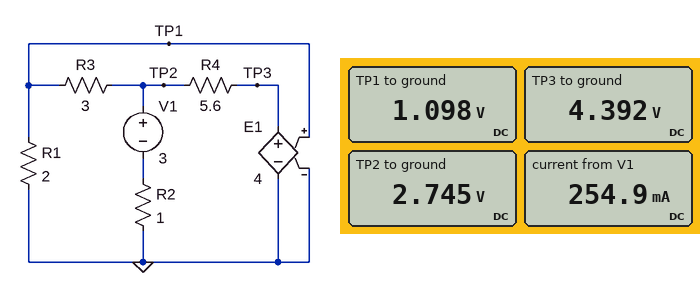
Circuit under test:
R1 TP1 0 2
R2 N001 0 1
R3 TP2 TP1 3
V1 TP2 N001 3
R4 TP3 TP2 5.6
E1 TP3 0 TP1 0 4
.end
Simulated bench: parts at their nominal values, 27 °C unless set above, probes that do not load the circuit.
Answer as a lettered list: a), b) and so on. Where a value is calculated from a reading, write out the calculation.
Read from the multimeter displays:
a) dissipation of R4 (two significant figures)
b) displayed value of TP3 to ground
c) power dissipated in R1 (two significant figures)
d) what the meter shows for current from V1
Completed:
a) (4.392 V - 2.745 V)^2 / 5.6 Ω = 480 mW
b) 4.392 V
c) (1.098 V)^2 / 2 Ω = 600 mW
d) 254.9 mA
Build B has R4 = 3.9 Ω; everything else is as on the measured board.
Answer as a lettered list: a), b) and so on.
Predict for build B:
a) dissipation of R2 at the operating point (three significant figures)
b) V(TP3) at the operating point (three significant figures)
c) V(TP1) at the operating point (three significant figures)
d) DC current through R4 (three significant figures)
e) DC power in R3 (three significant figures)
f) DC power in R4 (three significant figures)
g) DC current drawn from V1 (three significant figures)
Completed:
a) 17.5 mW
b) 4.59 V
c) 1.15 V
d) 441 mA
e) 987 mW
f) 759 mW
g) 132 mA
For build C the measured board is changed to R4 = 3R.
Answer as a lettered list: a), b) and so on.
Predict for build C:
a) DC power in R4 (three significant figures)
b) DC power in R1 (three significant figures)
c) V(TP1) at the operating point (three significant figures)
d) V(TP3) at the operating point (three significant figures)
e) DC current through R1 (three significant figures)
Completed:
a) 1.08 W
b) 720 mW
c) 1.20 V
d) 4.80 V
e) 600 mA
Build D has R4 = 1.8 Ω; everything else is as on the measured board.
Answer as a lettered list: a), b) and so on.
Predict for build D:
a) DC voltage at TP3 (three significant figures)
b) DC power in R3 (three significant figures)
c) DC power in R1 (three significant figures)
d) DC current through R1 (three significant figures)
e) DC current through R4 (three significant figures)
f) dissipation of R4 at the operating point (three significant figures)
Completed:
a) 5.54 V
b) 1.44 W
c) 959 mW
d) 692 mA
e) 1.15 A
f) 2.40 W
